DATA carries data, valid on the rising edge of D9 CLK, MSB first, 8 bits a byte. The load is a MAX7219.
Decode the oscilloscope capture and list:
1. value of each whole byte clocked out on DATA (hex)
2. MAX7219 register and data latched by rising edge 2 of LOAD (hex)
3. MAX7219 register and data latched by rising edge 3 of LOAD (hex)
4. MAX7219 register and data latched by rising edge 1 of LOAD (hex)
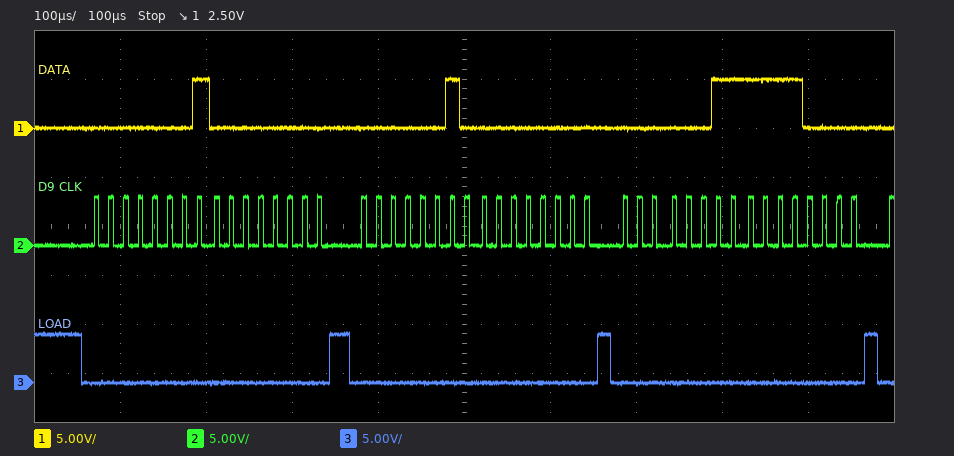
01 00 02 00 03 F0
register 0x2, data 0x00
register 0x3, data 0xF0
register 0x1, data 0x00
